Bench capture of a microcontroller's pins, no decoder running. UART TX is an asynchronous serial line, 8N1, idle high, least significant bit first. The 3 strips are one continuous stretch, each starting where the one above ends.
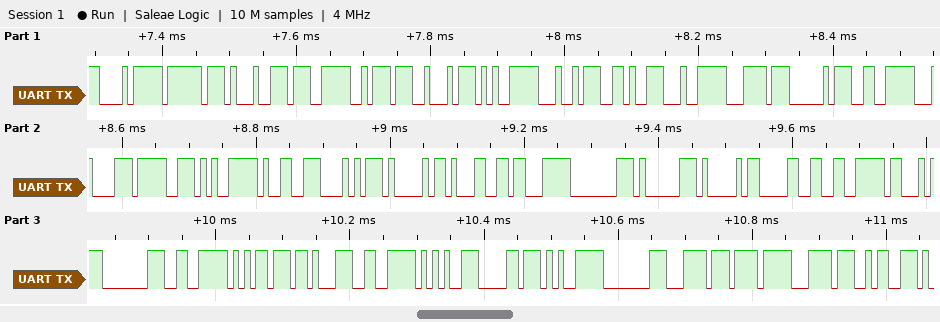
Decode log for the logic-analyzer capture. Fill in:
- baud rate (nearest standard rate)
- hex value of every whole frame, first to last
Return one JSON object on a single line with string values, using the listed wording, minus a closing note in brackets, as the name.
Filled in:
{"baud rate": "115200 baud", "hex value of every whole frame, first to last": "0xE8 0xBF 0x91 0xE7 0xBA 0xA2 0xE5 0xA4 0x96 0xE4 0xBC 0xA0 0xE6 0x84 0x9F 0xE5 0x99 0xA8 0x41 0x31 0xE3 0x80 0x81 0x41 0x30 0xE6 0xA3 0x80 0xE6 0xB5 0x8B 0xE6 0x95 0xB0 0xE5 0x80 0xBC 0xEF 0xBC 0x9A"}
